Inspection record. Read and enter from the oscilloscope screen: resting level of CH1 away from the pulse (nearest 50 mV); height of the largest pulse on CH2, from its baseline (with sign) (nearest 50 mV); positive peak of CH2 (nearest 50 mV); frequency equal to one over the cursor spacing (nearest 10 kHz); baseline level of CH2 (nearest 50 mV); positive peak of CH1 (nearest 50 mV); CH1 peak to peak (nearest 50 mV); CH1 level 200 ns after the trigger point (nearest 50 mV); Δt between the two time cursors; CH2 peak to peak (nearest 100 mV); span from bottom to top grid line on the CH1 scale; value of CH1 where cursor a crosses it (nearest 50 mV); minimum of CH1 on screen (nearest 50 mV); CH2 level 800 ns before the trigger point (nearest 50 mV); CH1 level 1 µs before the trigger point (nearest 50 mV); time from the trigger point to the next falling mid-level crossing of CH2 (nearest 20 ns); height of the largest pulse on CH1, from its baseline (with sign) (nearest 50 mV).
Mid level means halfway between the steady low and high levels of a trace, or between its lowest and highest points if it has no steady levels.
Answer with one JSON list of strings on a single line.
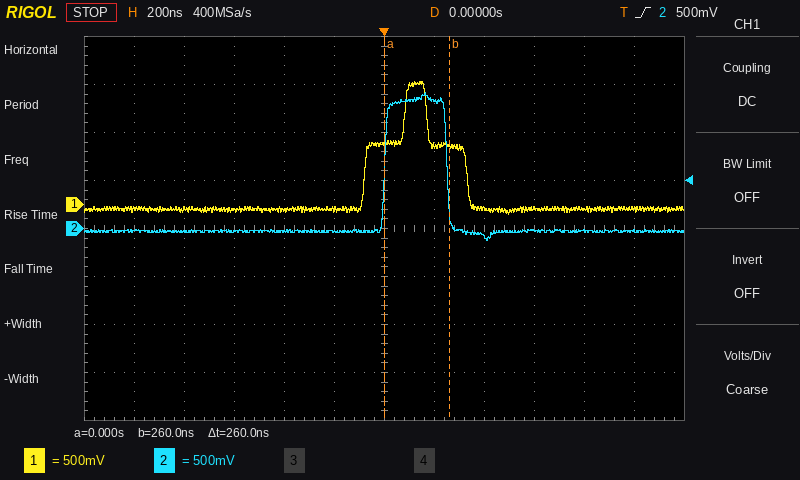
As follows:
["-50 mV", "+1.45 V", "1.40 V", "3.85 MHz", "-50 mV", "1.30 V", "1.40 V", "600 mV", "260 ns", "1.50 V", "4 V", "650 mV", "-100 mV", "-50 mV", "-50 mV", "260 ns", "+1.35 V"]
